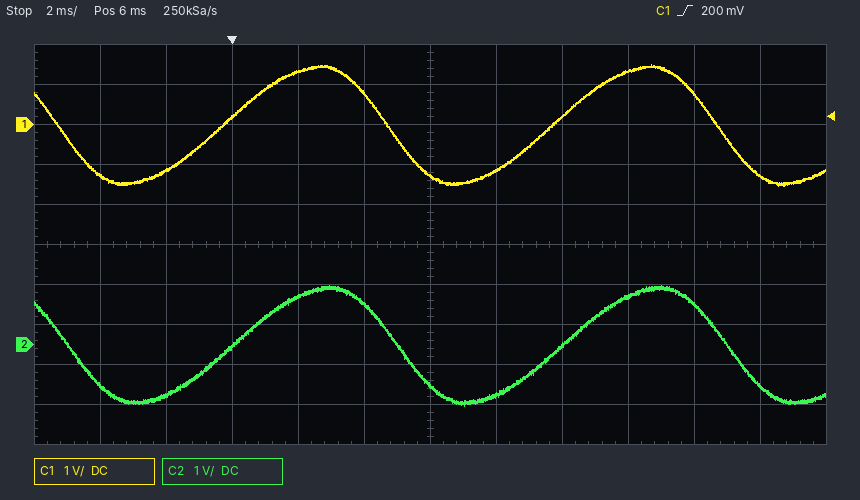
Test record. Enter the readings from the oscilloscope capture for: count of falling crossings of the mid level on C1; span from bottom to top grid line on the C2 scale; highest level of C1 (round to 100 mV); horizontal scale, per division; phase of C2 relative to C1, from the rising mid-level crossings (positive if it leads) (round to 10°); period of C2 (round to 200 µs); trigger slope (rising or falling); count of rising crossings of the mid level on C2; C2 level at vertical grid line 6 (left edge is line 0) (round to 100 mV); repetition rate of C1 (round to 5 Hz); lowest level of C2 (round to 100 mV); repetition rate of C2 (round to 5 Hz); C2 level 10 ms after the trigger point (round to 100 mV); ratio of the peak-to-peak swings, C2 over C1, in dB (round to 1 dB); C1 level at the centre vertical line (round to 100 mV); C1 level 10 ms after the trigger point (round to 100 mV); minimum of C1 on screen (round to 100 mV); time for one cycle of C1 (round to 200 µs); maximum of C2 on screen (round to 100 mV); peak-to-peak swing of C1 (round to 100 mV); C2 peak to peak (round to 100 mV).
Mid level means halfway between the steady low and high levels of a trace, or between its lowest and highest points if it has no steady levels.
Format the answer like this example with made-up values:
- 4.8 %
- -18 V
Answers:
- 3
- 10 V
- 1.5 V
- 2 ms
- -10°
- 10.0 ms
- rising
- 2
- -1.0 V
- 100 Hz
- -1.5 V
- 100 Hz
- 0.0 V
- 0 dB
- -1.3 V
- 200 mV
- -1.5 V
- 10.0 ms
- 1.5 V
- 3.0 V
- 3.0 V
